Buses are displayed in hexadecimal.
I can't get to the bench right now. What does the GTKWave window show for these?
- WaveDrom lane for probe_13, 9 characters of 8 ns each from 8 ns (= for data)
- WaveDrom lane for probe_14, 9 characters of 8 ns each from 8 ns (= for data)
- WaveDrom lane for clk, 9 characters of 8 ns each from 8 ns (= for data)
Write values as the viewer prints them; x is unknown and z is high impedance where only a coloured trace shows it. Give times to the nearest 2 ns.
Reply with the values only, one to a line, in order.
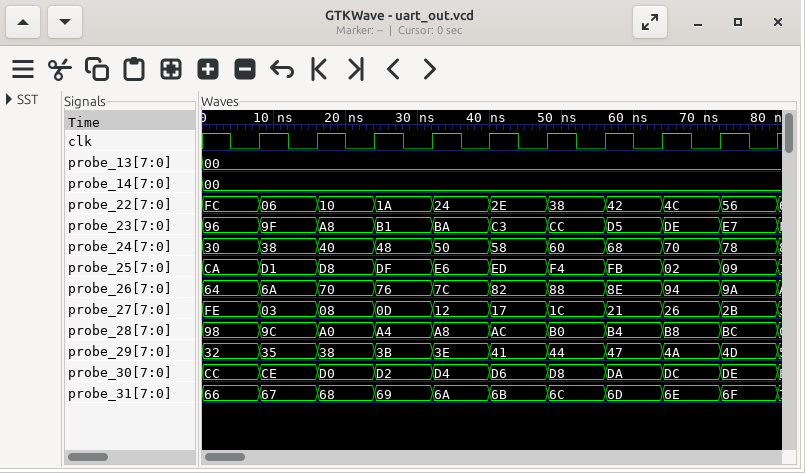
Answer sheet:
{name: 'probe_13', wave: '=........', data: '00'}
{name: 'probe_14', wave: '=........', data: '00'}
{name: 'clk', wave: 'p........'}
